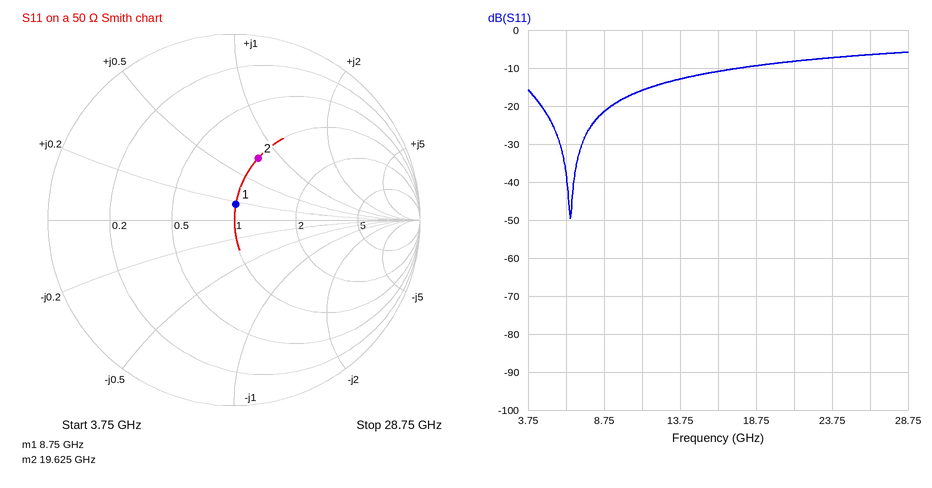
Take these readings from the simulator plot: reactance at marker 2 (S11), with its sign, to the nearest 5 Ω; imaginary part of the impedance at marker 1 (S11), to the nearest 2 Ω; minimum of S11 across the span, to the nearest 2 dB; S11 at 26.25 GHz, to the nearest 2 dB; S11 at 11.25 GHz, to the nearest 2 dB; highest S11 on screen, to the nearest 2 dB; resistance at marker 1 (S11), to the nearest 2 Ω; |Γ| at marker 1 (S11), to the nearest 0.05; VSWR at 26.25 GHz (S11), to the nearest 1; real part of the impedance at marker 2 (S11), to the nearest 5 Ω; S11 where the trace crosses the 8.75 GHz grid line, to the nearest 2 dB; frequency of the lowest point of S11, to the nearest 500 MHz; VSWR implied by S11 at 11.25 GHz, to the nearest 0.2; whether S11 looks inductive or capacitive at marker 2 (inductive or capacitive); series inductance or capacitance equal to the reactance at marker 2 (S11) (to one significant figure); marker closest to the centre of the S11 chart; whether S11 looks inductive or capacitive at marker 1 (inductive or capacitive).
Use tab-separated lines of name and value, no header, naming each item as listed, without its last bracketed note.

reactance at marker 2 (S11), with its sign, to the nearest 5 Ω	+40 Ω
imaginary part of the impedance at marker 1 (S11), to the nearest 2 Ω	+8 Ω
minimum of S11 across the span, to the nearest 2 dB	-50 dB
S11 at 26.25 GHz, to the nearest 2 dB	-6 dB
S11 at 11.25 GHz, to the nearest 2 dB	-16 dB
highest S11 on screen, to the nearest 2 dB	-6 dB
resistance at marker 1 (S11), to the nearest 2 Ω	50 Ω
|Γ| at marker 1 (S11), to the nearest 0.05	0.10
VSWR at 26.25 GHz (S11), to the nearest 1	3
real part of the impedance at marker 2 (S11), to the nearest 5 Ω	50 Ω
S11 where the trace crosses the 8.75 GHz grid line, to the nearest 2 dB	-22 dB
frequency of the lowest point of S11, to the nearest 500 MHz	6.5 GHz
VSWR implied by S11 at 11.25 GHz, to the nearest 0.2	1.4
whether S11 looks inductive or capacitive at marker 2	inductive
series inductance or capacitance equal to the reactance at marker 2 (S11)	300 pH
marker closest to the centre of the S11 chart	marker 1
whether S11 looks inductive or capacitive at marker 1	inductive
